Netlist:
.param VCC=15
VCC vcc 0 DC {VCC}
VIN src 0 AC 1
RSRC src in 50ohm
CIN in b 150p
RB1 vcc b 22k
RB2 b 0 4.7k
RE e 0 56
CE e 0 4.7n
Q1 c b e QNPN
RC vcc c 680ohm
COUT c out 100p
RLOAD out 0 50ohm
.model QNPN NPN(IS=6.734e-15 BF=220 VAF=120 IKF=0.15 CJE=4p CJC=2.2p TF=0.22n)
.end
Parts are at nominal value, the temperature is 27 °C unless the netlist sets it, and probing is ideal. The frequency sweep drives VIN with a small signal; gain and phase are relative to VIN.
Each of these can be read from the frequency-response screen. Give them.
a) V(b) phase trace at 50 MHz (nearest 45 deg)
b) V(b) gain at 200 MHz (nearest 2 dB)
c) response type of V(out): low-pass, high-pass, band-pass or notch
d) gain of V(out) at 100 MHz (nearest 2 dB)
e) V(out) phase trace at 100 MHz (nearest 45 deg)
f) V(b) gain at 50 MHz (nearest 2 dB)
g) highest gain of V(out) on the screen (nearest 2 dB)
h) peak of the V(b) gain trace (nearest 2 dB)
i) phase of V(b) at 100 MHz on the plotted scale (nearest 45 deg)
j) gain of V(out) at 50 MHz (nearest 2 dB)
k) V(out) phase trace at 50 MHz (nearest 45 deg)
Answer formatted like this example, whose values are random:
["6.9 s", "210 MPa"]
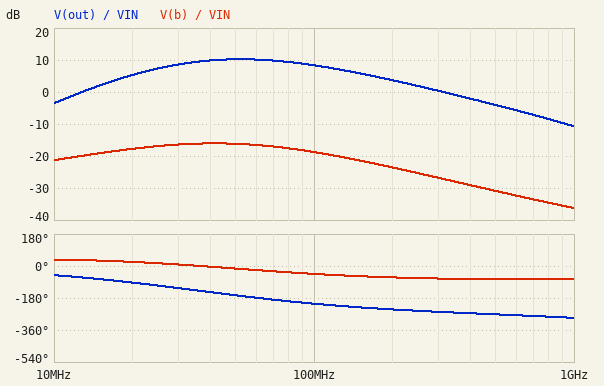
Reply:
["0 deg", "-24 dB", "band-pass", "8 dB", "-225 deg", "-16 dB", "10 dB", "-16 dB", "-45 deg", "10 dB", "-180 deg"]
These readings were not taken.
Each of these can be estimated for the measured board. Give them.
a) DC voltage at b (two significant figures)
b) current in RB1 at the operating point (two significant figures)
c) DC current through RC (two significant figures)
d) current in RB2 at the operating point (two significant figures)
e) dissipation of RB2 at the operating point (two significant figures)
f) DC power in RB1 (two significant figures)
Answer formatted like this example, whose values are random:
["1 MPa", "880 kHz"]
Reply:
["1.9 V", "600 µA", "20 mA", "400 µA", "760 µW", "7.8 mW"]
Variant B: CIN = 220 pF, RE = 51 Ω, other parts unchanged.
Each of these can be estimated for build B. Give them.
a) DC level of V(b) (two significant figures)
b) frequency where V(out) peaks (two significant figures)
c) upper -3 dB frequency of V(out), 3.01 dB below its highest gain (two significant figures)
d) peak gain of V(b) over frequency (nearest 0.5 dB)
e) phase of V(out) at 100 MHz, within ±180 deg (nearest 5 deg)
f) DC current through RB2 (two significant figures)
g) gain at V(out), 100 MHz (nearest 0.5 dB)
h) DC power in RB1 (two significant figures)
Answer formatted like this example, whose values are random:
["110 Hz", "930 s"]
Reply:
["1.8 V", "54 MHz", "130 MHz", "-16.5 dB", "150 deg", "380 µA", "7.5 dB", "7.9 mW"]
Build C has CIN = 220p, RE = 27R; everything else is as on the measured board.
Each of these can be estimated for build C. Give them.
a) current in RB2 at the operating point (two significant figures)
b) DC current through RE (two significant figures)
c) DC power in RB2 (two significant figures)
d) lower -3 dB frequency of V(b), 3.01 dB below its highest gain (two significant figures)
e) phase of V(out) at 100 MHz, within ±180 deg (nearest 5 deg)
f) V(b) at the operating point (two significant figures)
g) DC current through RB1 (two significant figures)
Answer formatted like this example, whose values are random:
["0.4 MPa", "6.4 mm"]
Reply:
["280 µA", "21 mA", "370 µW", "9.6 MHz", "165 deg", "1.3 V", "620 µA"]
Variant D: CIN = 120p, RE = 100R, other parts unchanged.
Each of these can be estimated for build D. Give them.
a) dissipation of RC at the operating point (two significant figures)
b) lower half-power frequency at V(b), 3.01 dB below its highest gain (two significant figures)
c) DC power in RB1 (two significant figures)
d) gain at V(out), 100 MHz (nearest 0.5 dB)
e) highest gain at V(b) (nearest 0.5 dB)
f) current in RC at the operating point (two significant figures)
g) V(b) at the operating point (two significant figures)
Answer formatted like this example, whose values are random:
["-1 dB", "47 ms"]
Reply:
["170 mW", "270 kHz", "7.3 mW", "13.0 dB", "-3.0 dB", "16 mA", "2.3 V"]
